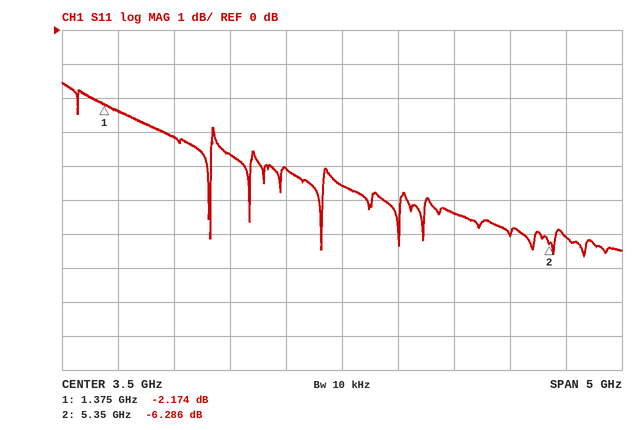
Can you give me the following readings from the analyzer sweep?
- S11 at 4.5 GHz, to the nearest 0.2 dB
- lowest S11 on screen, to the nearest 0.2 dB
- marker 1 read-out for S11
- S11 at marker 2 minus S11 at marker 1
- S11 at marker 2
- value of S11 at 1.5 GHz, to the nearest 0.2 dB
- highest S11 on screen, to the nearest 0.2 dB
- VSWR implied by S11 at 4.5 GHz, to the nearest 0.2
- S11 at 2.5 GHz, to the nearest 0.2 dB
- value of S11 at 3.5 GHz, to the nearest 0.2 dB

-5.4 dB
-6.6 dB
-2.174 dB
-4.112 dB
-6.286 dB
-2.4 dB
-1.6 dB
3.4
-3.6 dB
-4.6 dB
